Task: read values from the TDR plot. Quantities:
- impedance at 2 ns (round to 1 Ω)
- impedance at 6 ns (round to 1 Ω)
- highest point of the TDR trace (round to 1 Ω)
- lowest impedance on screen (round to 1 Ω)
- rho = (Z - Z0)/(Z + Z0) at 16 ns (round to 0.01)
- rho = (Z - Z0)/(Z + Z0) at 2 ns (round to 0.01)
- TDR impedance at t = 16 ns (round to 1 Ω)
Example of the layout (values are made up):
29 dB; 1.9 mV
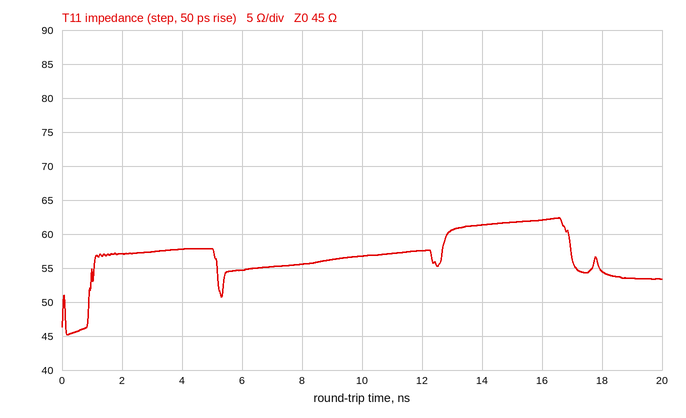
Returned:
57 Ω; 55 Ω; 62 Ω; 45 Ω; +0.16; +0.12; 62 Ω
